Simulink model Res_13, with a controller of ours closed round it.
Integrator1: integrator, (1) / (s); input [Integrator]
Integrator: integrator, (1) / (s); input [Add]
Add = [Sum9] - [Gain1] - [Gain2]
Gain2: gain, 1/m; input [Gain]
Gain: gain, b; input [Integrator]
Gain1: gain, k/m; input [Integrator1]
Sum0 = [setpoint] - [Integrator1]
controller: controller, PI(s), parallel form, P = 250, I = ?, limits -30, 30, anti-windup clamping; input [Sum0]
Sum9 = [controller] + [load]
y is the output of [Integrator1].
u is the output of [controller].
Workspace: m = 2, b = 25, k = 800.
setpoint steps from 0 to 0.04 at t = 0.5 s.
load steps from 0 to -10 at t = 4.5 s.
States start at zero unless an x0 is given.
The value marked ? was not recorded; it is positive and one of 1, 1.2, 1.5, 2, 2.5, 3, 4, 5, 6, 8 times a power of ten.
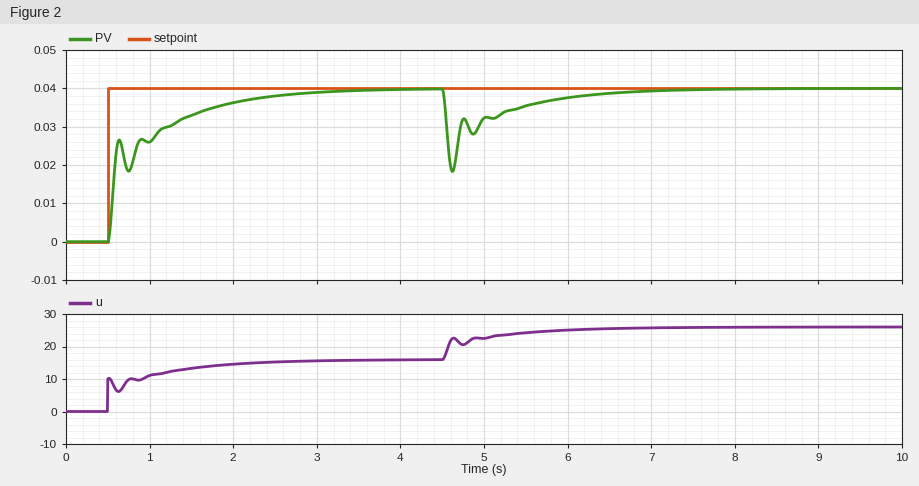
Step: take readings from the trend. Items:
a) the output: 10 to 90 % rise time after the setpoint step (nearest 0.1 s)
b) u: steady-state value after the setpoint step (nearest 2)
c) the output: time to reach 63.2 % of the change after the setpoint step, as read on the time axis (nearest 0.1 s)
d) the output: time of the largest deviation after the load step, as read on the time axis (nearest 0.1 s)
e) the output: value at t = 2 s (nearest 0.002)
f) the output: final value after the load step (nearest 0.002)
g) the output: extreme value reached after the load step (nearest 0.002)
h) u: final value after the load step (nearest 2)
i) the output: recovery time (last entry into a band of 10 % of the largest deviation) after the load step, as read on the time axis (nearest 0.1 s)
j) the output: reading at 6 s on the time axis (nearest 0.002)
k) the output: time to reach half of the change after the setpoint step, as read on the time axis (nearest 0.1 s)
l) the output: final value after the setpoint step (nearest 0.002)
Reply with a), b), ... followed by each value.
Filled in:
a) 1.4 s
b) 16
c) 0.6 s
d) 4.6 s
e) 0.036
f) 0.040
g) 0.018
h) 26
i) 6.1 s
j) 0.038
k) 0.6 s
l) 0.040
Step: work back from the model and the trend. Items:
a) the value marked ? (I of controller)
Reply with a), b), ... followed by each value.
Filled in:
a) 800
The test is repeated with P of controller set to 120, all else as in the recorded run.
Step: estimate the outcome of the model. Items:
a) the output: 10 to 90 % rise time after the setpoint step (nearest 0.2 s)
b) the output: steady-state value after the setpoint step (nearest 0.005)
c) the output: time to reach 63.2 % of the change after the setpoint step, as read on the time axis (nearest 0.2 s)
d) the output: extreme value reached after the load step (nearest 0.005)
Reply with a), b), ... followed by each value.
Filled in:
a) 1.2 s
b) 0.040
c) 1.0 s
d) 0.015
